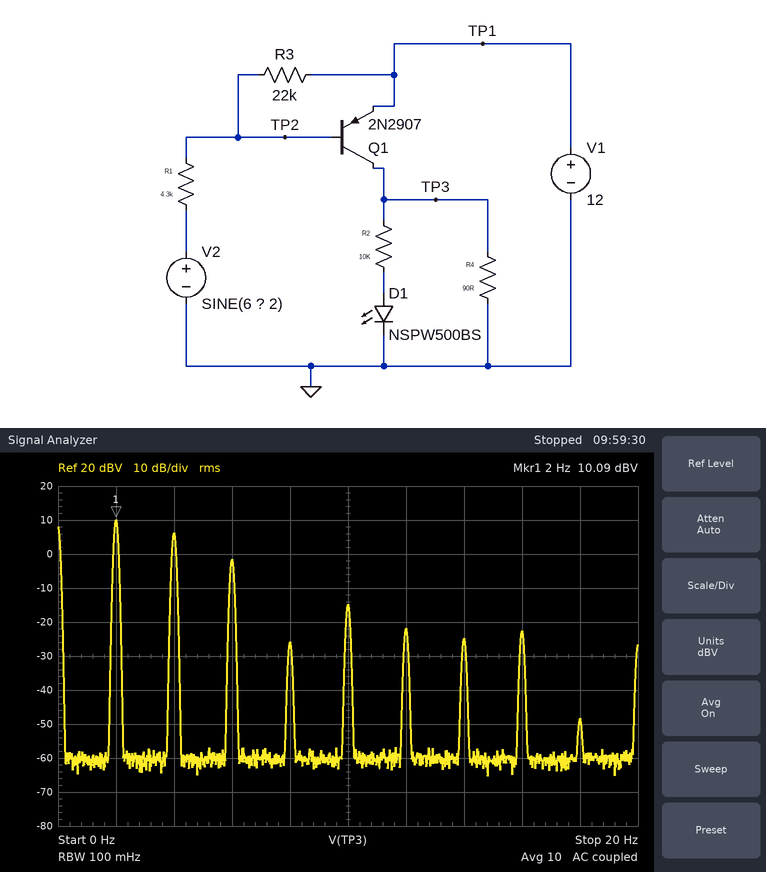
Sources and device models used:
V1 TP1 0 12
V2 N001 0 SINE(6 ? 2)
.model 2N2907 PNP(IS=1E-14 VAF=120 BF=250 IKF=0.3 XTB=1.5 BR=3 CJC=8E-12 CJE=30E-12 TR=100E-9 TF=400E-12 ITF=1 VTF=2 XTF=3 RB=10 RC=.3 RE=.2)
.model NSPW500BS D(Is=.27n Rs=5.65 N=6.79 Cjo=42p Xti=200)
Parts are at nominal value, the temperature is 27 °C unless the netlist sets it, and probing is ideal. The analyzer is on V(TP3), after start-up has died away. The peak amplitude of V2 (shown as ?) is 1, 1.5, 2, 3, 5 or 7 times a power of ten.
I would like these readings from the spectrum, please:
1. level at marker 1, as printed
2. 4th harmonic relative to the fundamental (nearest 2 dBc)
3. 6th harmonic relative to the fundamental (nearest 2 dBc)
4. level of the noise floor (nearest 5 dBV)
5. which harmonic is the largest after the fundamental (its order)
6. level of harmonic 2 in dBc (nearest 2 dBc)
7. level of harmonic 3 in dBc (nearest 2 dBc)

10.09 dBV
-36 dBc
-32 dBc
-60 dBV
2
-4 dBc
-12 dBc
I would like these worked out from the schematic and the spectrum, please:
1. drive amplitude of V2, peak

5 V
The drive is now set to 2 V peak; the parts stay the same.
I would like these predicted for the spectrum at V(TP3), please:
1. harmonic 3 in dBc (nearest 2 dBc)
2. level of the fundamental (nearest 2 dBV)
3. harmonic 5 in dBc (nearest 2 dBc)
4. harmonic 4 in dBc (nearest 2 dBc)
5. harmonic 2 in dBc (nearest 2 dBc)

-4 dBc
-18 dBV
-10 dBc
-6 dBc
-2 dBc
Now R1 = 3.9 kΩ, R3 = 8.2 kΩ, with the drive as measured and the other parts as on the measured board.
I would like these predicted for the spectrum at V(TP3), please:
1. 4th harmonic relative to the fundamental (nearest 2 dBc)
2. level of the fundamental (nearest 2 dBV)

-34 dBc
10 dBV
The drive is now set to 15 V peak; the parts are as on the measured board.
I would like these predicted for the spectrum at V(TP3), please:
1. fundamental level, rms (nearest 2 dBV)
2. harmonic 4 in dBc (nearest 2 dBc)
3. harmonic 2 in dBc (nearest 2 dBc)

14 dBV
-14 dBc
-12 dBc
